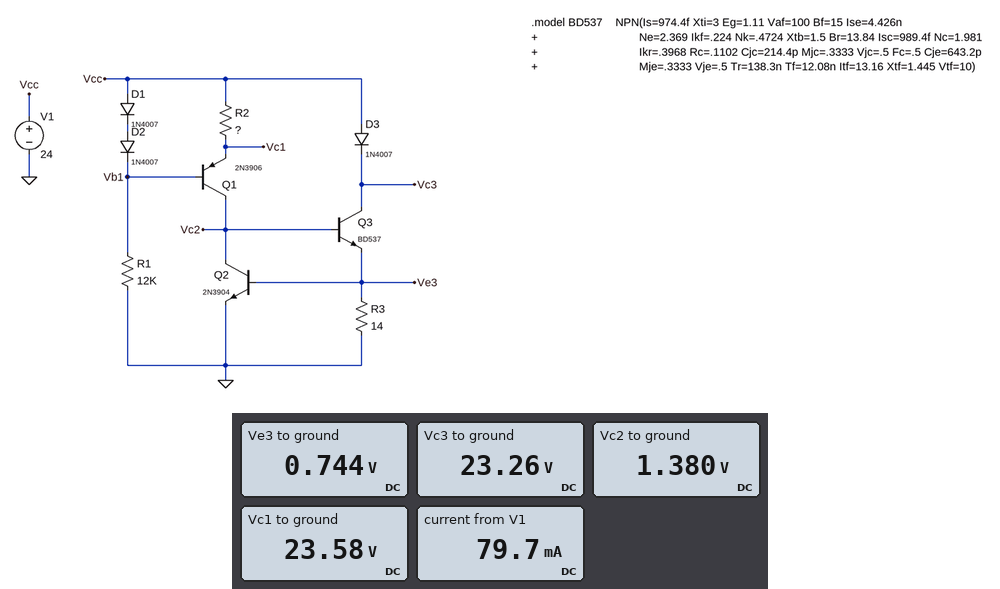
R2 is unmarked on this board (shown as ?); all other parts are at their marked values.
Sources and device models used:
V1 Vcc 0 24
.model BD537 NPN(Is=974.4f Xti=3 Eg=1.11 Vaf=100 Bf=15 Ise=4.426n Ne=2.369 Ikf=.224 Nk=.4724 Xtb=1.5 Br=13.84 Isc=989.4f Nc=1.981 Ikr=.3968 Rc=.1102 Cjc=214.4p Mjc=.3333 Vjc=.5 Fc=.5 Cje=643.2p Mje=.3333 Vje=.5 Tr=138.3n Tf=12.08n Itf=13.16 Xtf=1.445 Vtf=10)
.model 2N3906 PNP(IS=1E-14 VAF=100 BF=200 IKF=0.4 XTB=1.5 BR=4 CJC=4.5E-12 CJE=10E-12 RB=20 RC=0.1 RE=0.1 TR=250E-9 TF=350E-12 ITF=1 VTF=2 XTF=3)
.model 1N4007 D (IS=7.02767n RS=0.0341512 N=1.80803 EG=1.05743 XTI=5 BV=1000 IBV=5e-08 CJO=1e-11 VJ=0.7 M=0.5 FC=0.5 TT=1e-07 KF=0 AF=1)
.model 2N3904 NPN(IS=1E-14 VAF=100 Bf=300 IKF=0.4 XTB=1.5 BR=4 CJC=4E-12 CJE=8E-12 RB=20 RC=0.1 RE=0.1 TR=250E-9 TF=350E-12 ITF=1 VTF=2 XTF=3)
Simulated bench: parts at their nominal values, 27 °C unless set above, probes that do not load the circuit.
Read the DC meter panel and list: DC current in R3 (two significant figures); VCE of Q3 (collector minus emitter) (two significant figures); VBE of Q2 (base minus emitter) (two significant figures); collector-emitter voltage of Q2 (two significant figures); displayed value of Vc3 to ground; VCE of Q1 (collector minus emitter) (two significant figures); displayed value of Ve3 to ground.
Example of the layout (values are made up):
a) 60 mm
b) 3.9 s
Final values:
a) 53 mA
b) 23 V
c) 740 mV
d) 1.4 V
e) 23.26 V
f) -22 V
g) 0.744 V
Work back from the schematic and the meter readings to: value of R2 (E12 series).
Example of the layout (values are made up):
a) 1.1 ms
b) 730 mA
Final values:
a) 15 Ω
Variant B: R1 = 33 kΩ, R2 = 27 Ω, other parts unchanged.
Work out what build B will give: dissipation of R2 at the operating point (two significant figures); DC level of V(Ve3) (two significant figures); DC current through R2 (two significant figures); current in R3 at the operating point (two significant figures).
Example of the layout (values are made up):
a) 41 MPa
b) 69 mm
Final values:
a) 4.5 mW
b) 720 mV
c) 13 mA
d) 51 mA
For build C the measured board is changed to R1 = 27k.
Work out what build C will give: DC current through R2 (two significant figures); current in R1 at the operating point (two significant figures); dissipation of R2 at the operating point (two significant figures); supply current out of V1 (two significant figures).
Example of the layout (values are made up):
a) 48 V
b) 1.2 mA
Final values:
a) 23 mA
b) 850 µA
c) 8.0 mW
d) 73 mA
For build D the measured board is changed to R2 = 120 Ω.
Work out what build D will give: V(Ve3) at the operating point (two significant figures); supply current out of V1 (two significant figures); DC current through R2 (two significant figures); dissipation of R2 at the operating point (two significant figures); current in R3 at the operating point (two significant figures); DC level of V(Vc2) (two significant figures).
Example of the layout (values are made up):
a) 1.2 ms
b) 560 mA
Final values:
a) 660 mV
b) 50 mA
c) 4.0 mA
d) 1.9 mW
e) 47 mA
f) 1.3 V
